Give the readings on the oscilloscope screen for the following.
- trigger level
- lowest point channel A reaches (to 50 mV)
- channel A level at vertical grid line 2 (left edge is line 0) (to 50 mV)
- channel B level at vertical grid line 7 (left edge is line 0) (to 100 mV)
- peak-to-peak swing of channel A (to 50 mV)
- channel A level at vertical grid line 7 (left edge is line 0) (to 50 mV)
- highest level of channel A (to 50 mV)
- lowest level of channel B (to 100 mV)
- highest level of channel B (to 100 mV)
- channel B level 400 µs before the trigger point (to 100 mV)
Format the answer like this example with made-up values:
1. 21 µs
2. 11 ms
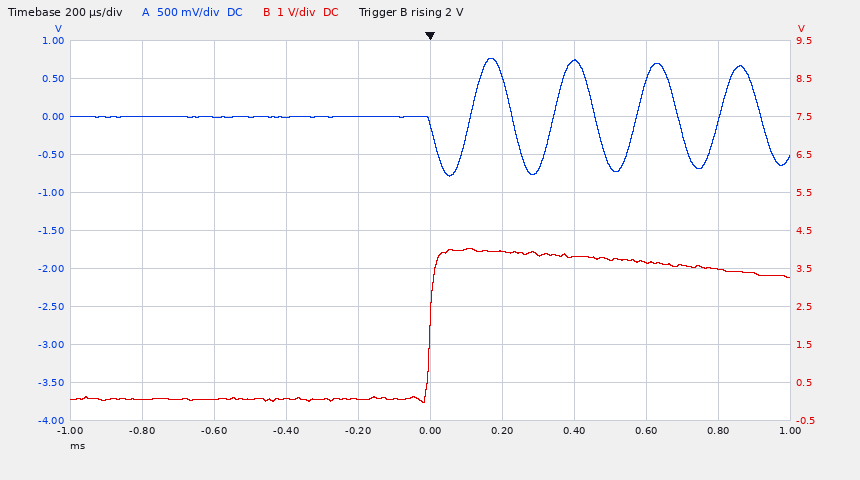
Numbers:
1. 2 V
2. -800 mV
3. 0 mV
4. 3.8 V
5. 1.55 V
6. 750 mV
7. 750 mV
8. 0.0 V
9. 4.0 V
10. 100 mV
